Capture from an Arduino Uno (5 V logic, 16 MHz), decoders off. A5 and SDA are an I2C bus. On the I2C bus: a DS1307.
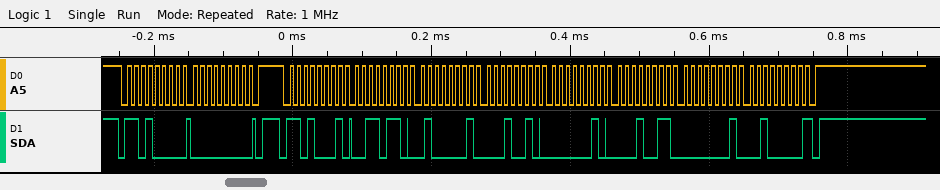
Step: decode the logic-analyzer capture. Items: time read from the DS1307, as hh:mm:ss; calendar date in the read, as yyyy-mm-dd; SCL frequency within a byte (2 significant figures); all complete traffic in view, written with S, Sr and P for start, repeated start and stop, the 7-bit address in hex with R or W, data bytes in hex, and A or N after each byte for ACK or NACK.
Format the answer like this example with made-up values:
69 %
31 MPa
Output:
12:41:36
2020-01-13
100 kHz
S 68W A 00 A P S 68R A 36 A 41 A 12 A 02 A 13 A 01 A 20 N P
